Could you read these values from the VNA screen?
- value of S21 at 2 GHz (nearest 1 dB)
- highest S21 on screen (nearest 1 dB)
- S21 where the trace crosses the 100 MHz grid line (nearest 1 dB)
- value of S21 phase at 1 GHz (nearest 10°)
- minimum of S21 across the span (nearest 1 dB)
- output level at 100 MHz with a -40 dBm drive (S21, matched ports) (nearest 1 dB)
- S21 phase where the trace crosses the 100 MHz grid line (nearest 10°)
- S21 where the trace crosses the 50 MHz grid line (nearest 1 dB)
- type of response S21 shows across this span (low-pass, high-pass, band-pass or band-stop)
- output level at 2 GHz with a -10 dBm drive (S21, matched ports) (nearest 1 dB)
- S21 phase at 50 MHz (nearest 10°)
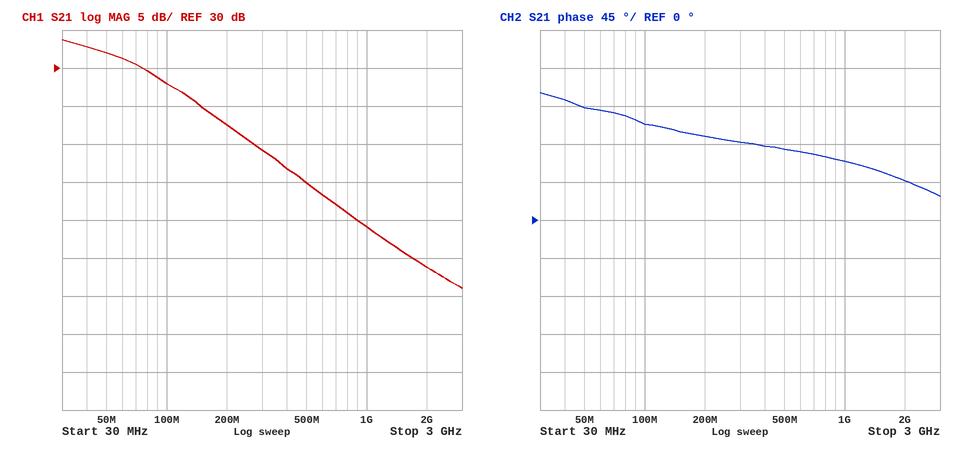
4 dB
34 dB
28 dB
70°
1 dB
-12 dBm
110°
32 dB
low-pass
-6 dBm
130°
